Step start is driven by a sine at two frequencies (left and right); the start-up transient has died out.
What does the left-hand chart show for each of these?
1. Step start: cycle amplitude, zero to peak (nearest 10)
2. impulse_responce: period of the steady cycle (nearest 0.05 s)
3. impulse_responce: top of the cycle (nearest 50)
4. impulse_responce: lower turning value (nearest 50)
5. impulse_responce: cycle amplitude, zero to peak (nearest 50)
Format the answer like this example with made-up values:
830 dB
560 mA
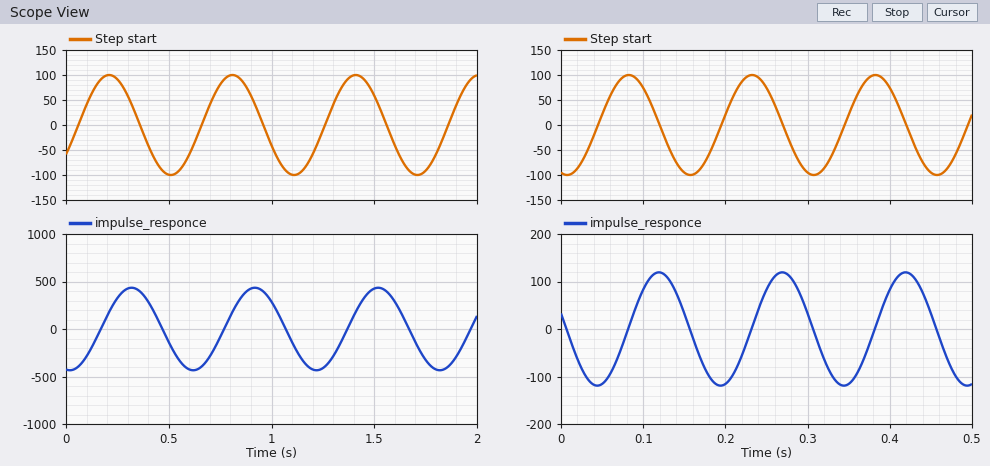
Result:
100
0.60 s
450
-450
450
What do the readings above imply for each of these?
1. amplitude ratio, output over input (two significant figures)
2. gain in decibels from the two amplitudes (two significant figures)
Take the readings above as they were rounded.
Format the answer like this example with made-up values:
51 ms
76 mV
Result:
4.5
13 dB
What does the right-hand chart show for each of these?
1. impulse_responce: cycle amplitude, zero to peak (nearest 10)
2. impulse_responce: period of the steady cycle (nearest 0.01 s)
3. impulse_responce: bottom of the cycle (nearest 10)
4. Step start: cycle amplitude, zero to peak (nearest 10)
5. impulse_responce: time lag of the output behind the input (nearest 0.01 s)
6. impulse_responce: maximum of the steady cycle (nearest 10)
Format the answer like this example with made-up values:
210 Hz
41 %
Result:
120
0.15 s
-120
100
0.04 s
120
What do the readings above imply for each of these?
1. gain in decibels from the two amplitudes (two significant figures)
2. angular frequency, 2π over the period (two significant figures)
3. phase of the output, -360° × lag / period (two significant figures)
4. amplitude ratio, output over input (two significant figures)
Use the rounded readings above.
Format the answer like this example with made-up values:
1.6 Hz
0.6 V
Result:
1.6 dB
42 rad/s
-96°
1.2
